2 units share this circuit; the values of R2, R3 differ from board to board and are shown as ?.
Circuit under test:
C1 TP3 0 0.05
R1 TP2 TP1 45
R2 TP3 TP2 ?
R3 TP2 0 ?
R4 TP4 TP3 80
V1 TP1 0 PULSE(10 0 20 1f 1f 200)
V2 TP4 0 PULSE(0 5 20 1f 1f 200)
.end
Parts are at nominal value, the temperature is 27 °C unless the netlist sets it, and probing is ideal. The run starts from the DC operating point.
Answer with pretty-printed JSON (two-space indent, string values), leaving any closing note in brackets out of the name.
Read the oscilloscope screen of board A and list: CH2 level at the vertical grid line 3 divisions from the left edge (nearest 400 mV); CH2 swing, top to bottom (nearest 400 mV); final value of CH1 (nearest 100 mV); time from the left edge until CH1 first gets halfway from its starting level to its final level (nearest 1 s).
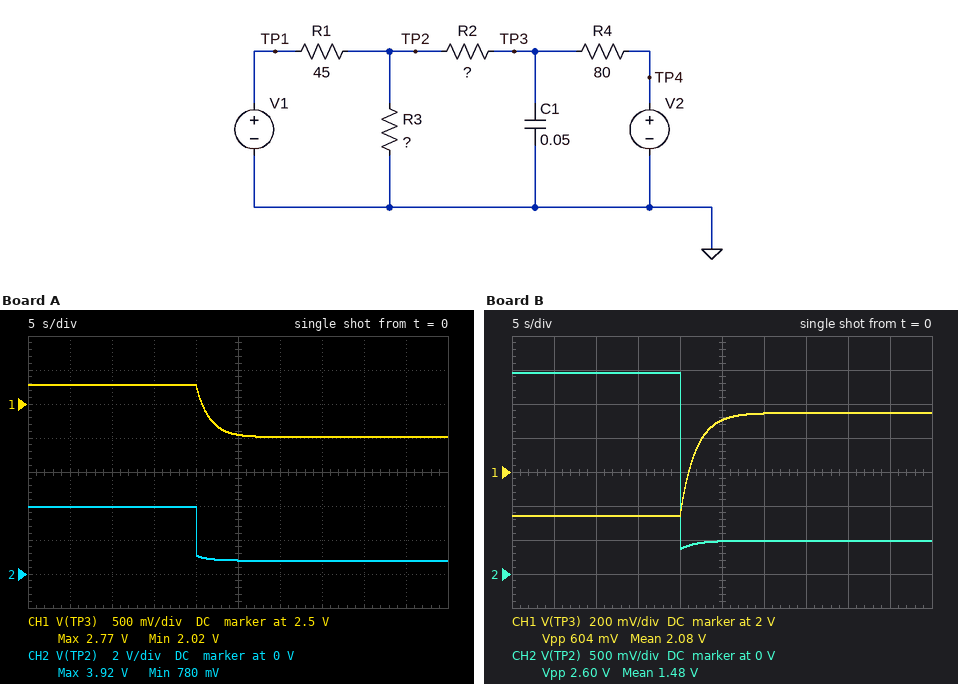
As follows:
{
  "CH2 level at the vertical grid line 3 divisions from the left edge": "4.0 V",
  "CH2 swing, top to bottom": "3.2 V",
  "final value of CH1": "2.0 V",
  "time from the left edge until CH1 first gets halfway from its starting level to its final level": "21 s"
}
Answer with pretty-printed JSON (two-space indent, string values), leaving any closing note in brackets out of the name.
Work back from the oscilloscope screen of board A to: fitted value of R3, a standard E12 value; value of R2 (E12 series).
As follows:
{
  "fitted value of R3, a standard E12 value": "39 Ω",
  "value of R2": "33 Ω"
}
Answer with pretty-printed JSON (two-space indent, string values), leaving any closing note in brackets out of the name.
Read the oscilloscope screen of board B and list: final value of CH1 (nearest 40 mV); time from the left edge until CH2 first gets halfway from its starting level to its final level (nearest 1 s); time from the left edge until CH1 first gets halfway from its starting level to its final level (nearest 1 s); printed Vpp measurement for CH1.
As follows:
{
  "final value of CH1": "2.36 V",
  "time from the left edge until CH2 first gets halfway from its starting level to its final level": "20 s",
  "time from the left edge until CH1 first gets halfway from its starting level to its final level": "21 s",
  "printed Vpp measurement for CH1": "604 mV"
}
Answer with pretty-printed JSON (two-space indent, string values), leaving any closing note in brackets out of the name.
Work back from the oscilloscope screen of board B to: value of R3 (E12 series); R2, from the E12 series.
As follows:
{
  "value of R3": "22 Ω",
  "R2, from the E12 series": "56 Ω"
}
